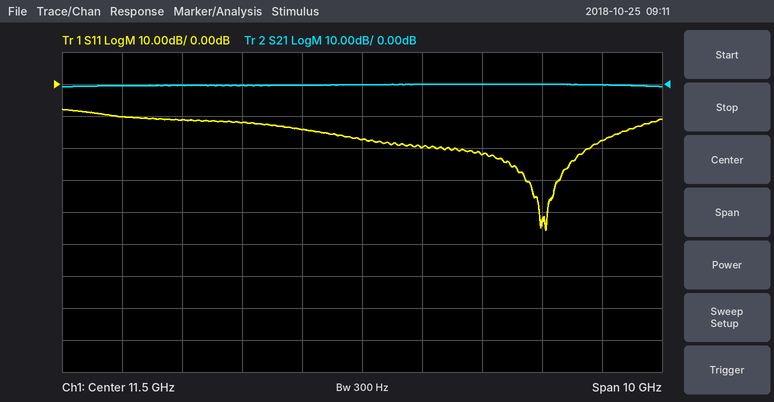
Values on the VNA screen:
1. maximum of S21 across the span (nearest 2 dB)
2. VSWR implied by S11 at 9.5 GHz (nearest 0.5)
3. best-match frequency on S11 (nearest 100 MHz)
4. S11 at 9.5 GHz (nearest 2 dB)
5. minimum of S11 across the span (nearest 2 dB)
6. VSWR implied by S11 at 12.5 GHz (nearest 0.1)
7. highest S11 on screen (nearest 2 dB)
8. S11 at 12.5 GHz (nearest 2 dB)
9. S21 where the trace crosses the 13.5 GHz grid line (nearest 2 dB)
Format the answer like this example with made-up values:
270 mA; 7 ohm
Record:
0 dB; 1.5; 14.6 GHz; -12 dB; -46 dB; 1.2; -8 dB; -20 dB; 0 dB
